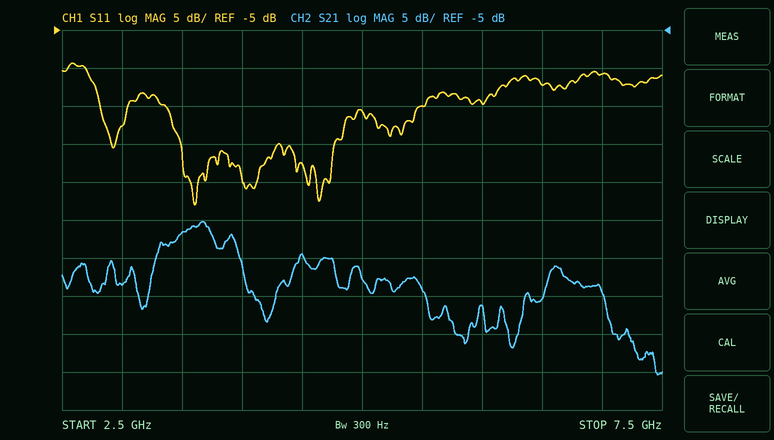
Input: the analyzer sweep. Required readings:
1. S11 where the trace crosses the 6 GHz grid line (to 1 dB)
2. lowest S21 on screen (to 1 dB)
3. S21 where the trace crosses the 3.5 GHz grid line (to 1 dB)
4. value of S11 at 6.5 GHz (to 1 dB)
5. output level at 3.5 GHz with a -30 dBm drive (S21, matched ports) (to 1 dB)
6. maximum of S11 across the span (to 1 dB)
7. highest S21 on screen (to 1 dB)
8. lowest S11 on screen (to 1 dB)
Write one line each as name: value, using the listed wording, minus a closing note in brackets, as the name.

S11 where the trace crosses the 6 GHz grid line: -15 dB
lowest S21 on screen: -50 dB
S21 where the trace crosses the 3.5 GHz grid line: -32 dB
value of S11 at 6.5 GHz: -12 dB
output level at 3.5 GHz with a -30 dBm drive (S21, matched ports): -62 dBm
maximum of S11 across the span: -9 dB
highest S21 on screen: -30 dB
lowest S11 on screen: -28 dB
